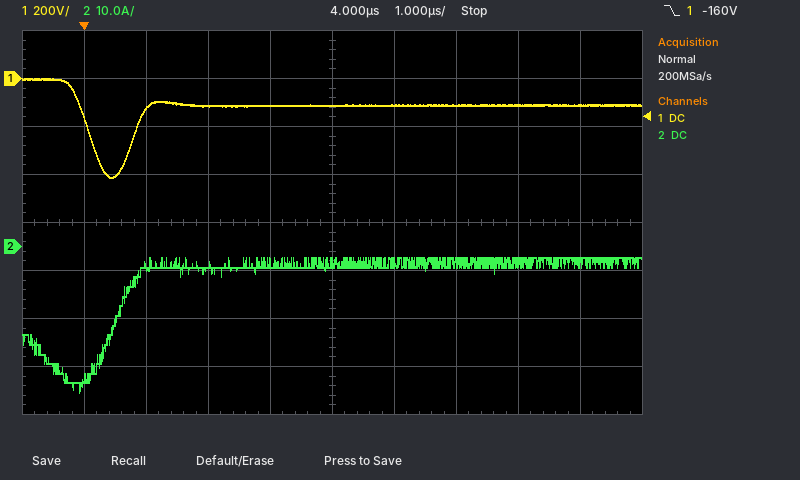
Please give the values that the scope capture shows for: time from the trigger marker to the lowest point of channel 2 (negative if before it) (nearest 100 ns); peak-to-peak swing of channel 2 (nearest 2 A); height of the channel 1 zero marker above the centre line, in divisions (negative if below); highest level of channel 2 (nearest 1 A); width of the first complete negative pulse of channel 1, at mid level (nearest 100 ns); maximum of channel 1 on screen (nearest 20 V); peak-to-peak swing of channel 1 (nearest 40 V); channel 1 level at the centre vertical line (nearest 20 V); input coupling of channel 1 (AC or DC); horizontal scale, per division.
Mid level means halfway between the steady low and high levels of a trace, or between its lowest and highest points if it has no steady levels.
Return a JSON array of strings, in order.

["-100 ns", "28 A", "+3.0 div", "-2 A", "800 ns", "0 V", "400 V", "-120 V", "DC", "1 µs"]
